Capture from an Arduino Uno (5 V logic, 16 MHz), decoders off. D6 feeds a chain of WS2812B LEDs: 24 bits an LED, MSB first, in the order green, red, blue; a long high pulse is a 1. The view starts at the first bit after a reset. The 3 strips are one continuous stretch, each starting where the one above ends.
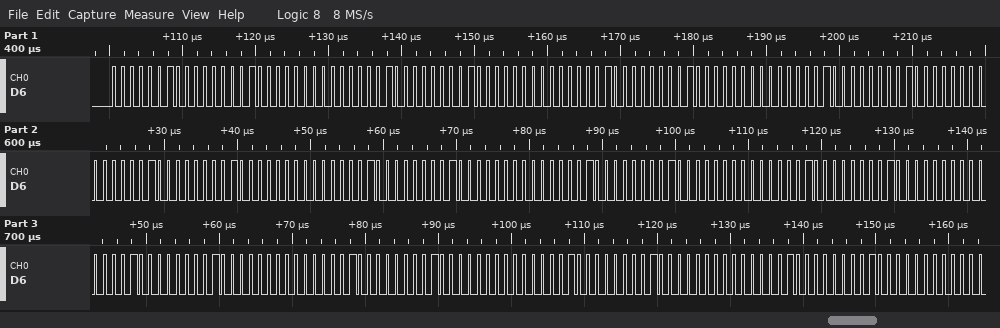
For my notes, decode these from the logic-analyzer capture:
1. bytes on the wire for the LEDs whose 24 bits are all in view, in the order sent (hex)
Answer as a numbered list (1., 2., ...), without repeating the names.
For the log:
1. 02 01 00 02 01 00 02 01 00 02 01 00 02 01 00 02 01 00 02 01 00 02 01 00 02 01 00 02 01 00 02 01 00 02 01 00
